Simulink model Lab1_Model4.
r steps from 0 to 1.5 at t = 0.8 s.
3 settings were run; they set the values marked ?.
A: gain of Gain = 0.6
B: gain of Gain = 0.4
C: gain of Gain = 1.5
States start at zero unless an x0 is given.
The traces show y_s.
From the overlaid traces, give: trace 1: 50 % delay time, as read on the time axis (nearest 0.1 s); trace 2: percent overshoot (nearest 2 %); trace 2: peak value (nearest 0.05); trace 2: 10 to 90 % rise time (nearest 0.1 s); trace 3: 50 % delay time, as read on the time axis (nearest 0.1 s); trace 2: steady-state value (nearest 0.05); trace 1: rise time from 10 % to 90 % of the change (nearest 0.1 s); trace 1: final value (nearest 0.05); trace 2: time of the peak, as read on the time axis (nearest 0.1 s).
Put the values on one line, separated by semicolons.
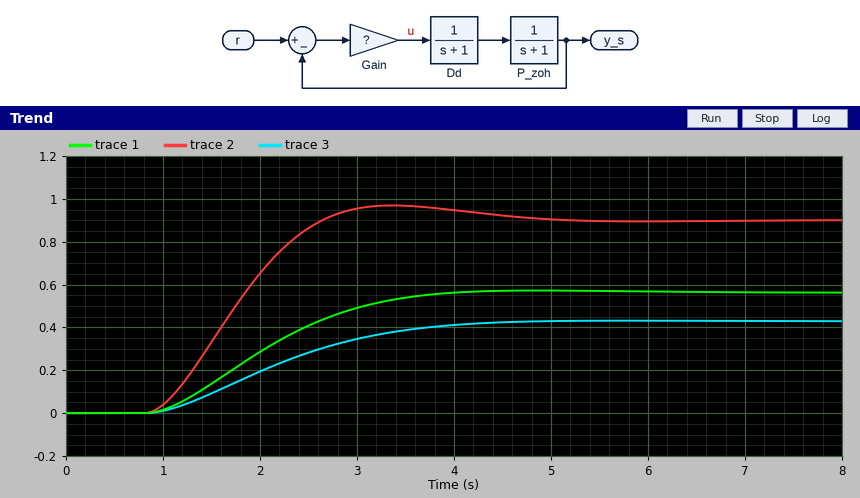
2.0 s; 8 %; 0.95; 1.2 s; 2.1 s; 0.90; 1.9 s; 0.55; 3.4 s
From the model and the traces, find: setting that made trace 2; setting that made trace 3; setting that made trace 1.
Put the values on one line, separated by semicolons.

C; B; A
